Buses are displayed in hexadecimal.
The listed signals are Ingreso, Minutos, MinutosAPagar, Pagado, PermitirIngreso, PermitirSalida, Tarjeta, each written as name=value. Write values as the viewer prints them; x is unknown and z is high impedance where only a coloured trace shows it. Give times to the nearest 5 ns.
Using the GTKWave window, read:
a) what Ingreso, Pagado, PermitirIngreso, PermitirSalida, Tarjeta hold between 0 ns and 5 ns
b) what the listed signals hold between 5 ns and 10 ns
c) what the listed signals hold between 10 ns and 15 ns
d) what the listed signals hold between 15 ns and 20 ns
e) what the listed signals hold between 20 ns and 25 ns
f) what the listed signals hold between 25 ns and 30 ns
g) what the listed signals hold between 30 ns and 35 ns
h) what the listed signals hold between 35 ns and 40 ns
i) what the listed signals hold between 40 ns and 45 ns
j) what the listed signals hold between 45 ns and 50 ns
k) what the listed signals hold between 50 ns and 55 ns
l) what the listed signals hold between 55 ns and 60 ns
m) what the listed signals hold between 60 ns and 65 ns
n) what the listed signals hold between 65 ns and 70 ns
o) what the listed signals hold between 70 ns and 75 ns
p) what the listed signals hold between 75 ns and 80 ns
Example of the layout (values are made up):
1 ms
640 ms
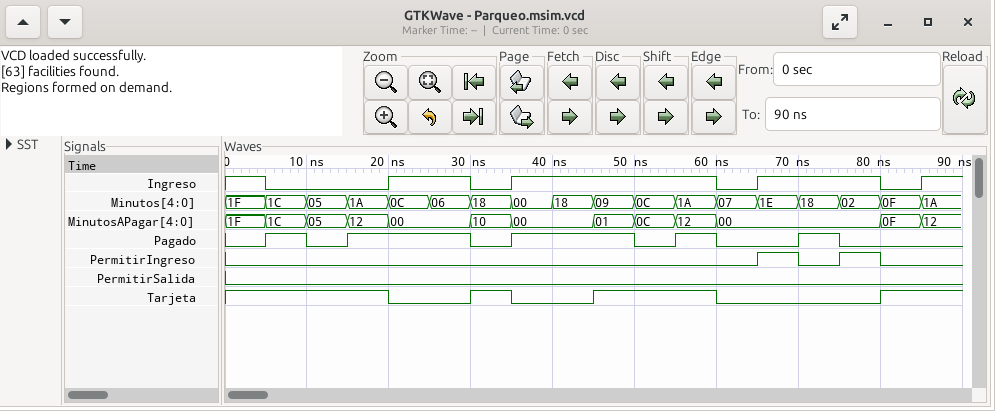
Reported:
Ingreso=1, Pagado=0, PermitirIngreso=0, PermitirSalida=0, Tarjeta=1
Ingreso=0, Minutos=1C, MinutosAPagar=1C, Pagado=1, PermitirIngreso=0, PermitirSalida=0, Tarjeta=1
Ingreso=0, Minutos=05, MinutosAPagar=05, Pagado=0, PermitirIngreso=0, PermitirSalida=0, Tarjeta=1
Ingreso=0, Minutos=1A, MinutosAPagar=12, Pagado=1, PermitirIngreso=0, PermitirSalida=0, Tarjeta=1
Ingreso=1, Minutos=0C, MinutosAPagar=00, Pagado=1, PermitirIngreso=0, PermitirSalida=0, Tarjeta=0
Ingreso=1, Minutos=06, MinutosAPagar=00, Pagado=1, PermitirIngreso=0, PermitirSalida=0, Tarjeta=0
Ingreso=0, Minutos=18, MinutosAPagar=10, Pagado=0, PermitirIngreso=0, PermitirSalida=0, Tarjeta=1
Ingreso=1, Minutos=00, MinutosAPagar=00, Pagado=1, PermitirIngreso=0, PermitirSalida=0, Tarjeta=0
Ingreso=1, Minutos=18, MinutosAPagar=00, Pagado=1, PermitirIngreso=0, PermitirSalida=0, Tarjeta=0
Ingreso=1, Minutos=09, MinutosAPagar=01, Pagado=1, PermitirIngreso=0, PermitirSalida=0, Tarjeta=1
Ingreso=1, Minutos=0C, MinutosAPagar=0C, Pagado=0, PermitirIngreso=0, PermitirSalida=0, Tarjeta=1
Ingreso=1, Minutos=1A, MinutosAPagar=12, Pagado=1, PermitirIngreso=0, PermitirSalida=0, Tarjeta=1
Ingreso=0, Minutos=07, MinutosAPagar=00, Pagado=0, PermitirIngreso=0, PermitirSalida=0, Tarjeta=0
Ingreso=1, Minutos=1E, MinutosAPagar=00, Pagado=0, PermitirIngreso=1, PermitirSalida=0, Tarjeta=0
Ingreso=1, Minutos=18, MinutosAPagar=00, Pagado=1, PermitirIngreso=0, PermitirSalida=0, Tarjeta=0
Ingreso=1, Minutos=02, MinutosAPagar=00, Pagado=0, PermitirIngreso=1, PermitirSalida=0, Tarjeta=0
